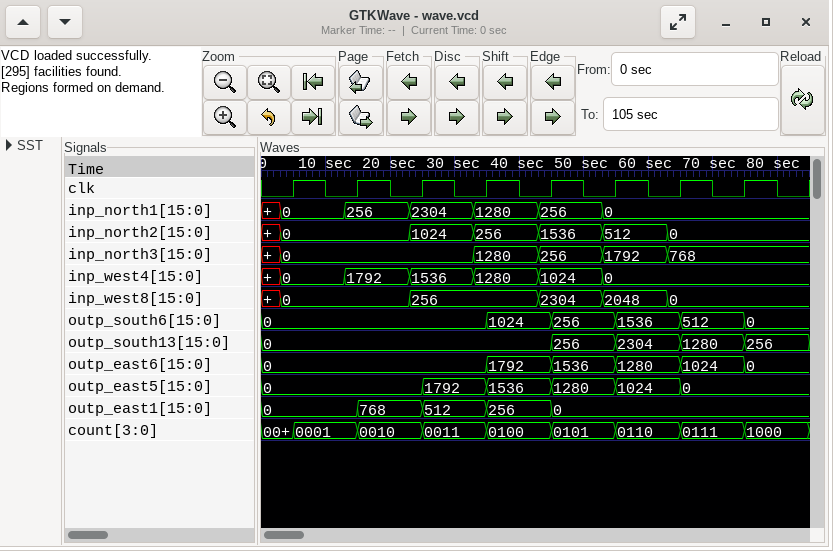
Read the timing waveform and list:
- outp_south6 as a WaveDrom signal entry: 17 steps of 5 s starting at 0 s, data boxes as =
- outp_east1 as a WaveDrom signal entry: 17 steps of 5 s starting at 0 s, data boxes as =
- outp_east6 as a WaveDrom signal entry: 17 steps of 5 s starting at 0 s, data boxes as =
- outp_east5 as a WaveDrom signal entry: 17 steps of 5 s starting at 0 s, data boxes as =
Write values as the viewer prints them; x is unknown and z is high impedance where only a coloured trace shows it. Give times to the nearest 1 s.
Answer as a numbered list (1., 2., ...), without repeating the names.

1. {name: 'outp_south6', wave: '=......=.=.=.=.=.', data: '0 1024 256 1536 512 0'}
2. {name: 'outp_east1', wave: '=..=.=.=.=.......', data: '0 768 512 256 0'}
3. {name: 'outp_east6', wave: '=......=.=.=.=.=.', data: '0 1792 1536 1280 1024 0'}
4. {name: 'outp_east5', wave: '=....=.=.=.=.=...', data: '0 1792 1536 1280 1024 0'}
